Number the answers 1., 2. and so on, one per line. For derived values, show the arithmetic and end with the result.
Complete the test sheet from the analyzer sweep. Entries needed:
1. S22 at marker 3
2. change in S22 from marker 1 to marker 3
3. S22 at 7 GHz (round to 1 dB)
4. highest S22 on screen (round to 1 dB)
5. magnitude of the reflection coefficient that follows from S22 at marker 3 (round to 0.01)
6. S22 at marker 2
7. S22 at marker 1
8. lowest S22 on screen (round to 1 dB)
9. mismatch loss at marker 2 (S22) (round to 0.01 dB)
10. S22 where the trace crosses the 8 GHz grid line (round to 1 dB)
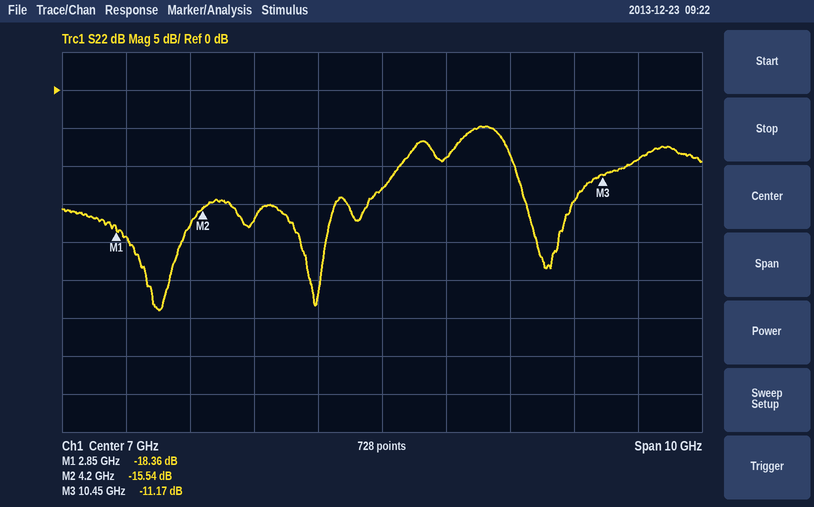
1. -11.17 dB
2. -11.17 − (-18.36) = 7.19 dB
3. -13 dB
4. -5 dB
5. 10^(-11.17/20) ≈ 0.28
6. -15.54 dB
7. -18.36 dB
8. -29 dB
9. −10 log10(1 − 10^(-15.54/10)) ≈ 0.12 dB
10. -9 dB
